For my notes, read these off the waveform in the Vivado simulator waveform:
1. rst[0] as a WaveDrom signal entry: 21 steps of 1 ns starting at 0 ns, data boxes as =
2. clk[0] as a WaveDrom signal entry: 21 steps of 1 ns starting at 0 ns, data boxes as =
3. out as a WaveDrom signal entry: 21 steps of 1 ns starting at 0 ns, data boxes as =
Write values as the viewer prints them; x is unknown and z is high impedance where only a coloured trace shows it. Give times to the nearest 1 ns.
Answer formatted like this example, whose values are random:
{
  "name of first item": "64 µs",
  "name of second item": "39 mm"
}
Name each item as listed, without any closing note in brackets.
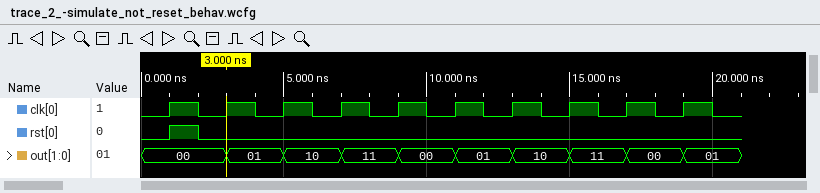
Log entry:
{
  "rst[0] as a WaveDrom signal entry: 21 steps of 1 ns starting at 0 ns, data boxes as =": "{name: 'rst[0]', wave: '010..................'}",
  "clk[0] as a WaveDrom signal entry: 21 steps of 1 ns starting at 0 ns, data boxes as =": "{name: 'clk[0]', wave: '010101010101010101010'}",
  "out as a WaveDrom signal entry: 21 steps of 1 ns starting at 0 ns, data boxes as =": "{name: 'out', wave: '=..=.=.=.=.=.=.=.=.=.', data: '00 01 10 11 00 01 10 11 00 01'}"
}
